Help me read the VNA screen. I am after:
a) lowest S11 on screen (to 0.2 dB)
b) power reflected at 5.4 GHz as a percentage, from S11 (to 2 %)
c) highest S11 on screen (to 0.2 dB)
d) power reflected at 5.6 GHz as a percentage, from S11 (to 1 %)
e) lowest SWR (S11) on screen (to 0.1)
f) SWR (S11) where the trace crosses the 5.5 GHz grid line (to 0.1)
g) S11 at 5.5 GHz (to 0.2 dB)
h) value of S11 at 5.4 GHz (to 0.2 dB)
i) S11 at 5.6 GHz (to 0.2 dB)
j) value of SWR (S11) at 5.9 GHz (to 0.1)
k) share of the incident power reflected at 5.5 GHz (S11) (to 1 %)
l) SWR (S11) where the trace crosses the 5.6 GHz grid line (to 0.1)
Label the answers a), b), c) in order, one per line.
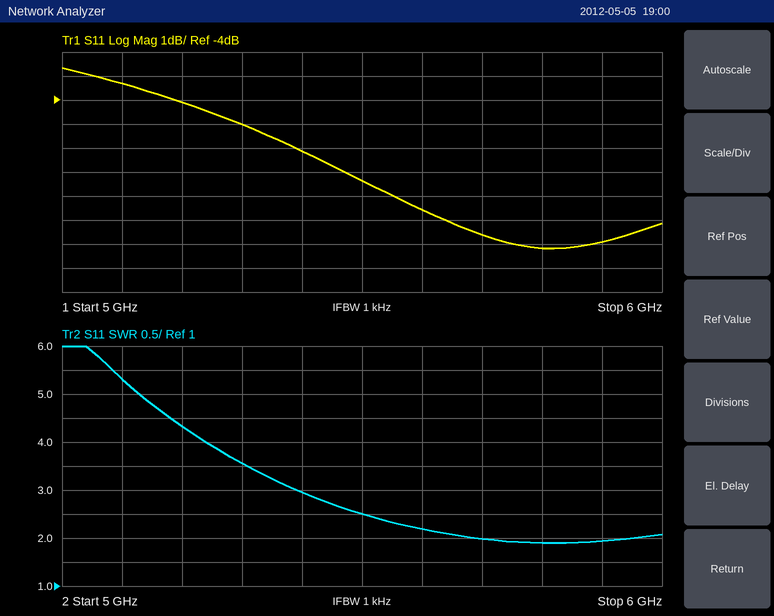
a) -10.2 dB
b) 24 %
c) -2.6 dB
d) 14 %
e) 1.9
f) 2.5
g) -7.4 dB
h) -6.2 dB
i) -8.6 dB
j) 1.9
k) 18 %
l) 2.2
